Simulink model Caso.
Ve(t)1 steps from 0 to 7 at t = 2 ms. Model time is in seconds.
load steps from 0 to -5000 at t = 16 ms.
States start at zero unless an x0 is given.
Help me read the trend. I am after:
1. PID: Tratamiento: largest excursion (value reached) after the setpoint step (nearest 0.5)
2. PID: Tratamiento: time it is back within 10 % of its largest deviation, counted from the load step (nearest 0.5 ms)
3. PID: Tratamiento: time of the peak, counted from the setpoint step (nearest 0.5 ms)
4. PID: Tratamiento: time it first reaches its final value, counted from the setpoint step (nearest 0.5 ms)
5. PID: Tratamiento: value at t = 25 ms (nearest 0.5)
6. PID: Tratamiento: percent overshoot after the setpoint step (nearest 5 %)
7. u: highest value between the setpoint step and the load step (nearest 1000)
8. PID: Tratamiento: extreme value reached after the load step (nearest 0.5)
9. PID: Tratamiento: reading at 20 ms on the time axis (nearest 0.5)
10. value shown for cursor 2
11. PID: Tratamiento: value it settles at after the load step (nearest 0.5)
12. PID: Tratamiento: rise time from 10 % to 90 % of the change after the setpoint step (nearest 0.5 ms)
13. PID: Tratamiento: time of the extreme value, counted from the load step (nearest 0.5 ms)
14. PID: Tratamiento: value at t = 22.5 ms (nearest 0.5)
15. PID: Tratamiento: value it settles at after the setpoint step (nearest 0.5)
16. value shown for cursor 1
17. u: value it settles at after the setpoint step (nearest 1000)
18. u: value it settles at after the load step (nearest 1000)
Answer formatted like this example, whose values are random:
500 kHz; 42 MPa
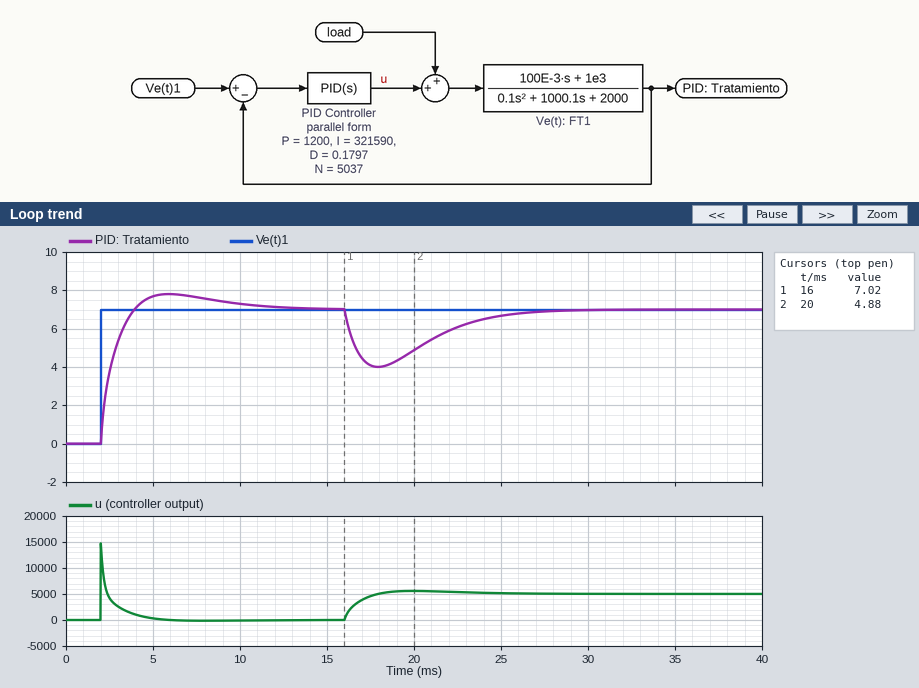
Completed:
8.0; 9.0 ms; 4.0 ms; 2.0 ms; 6.5; 10 %; 15000; 4.0; 5.0; 4.88; 7.0; 1.5 ms; 2.0 ms; 6.0; 7.0; 7.02; 0; 5000
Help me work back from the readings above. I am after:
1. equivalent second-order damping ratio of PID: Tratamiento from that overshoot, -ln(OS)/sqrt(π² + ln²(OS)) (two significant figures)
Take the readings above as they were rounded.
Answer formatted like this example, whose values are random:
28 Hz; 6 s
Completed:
0.59
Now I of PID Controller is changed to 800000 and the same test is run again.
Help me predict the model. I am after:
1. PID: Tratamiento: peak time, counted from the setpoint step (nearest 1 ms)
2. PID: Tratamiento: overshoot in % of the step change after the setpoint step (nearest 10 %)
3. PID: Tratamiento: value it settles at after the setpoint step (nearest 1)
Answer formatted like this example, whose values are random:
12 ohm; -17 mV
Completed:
3 ms; 20 %; 7
